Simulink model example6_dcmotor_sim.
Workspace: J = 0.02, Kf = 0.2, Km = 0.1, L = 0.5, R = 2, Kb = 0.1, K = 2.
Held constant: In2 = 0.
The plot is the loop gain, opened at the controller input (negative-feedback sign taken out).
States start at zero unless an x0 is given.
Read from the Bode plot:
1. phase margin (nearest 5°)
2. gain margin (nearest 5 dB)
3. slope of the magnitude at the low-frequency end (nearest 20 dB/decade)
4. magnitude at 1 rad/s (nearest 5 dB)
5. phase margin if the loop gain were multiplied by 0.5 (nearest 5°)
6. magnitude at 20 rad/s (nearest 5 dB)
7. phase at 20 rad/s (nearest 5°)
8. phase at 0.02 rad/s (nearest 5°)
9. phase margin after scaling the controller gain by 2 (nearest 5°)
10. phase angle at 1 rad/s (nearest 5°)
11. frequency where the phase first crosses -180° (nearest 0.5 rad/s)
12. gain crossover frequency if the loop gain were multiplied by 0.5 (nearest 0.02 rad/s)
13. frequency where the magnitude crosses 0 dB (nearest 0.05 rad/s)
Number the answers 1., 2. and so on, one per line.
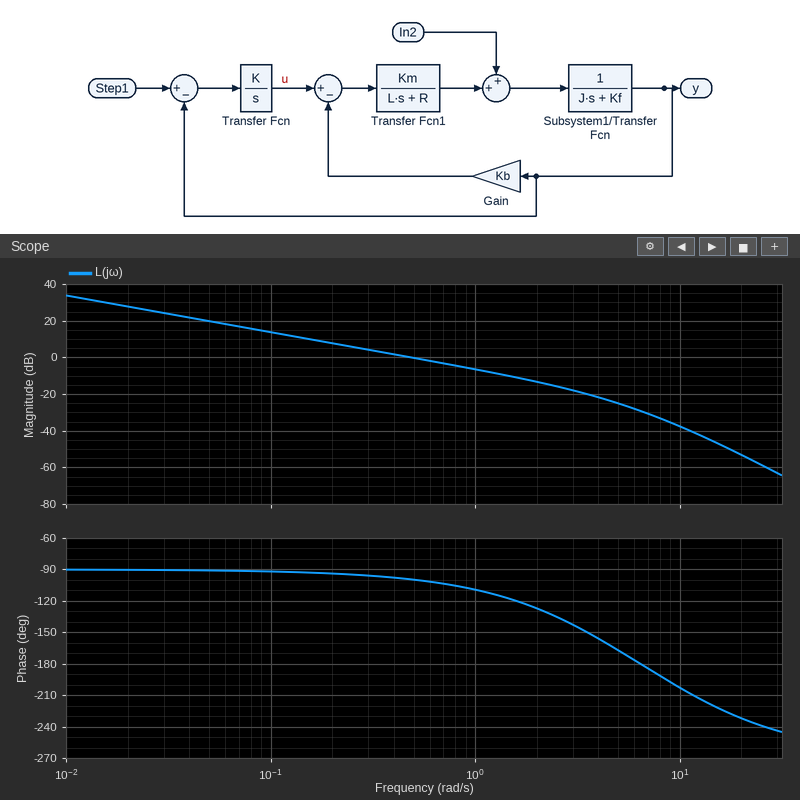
1. 80°
2. 30 dB
3. -20 dB/decade
4. -5 dB
5. 85°
6. -55 dB
7. -230°
8. -90°
9. 70°
10. -110°
11. 6.5 rad/s
12. 0.24 rad/s
13. 0.50 rad/s
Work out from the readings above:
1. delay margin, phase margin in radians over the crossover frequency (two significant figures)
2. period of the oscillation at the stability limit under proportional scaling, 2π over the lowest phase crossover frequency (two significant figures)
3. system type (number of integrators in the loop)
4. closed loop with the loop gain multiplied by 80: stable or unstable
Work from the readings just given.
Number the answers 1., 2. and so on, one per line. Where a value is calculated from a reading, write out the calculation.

1. 80 × π / 180 / 0.5 = 2.8 s
2. 2π / 6.5 = 0.97 s
3. 1
4. unstable
